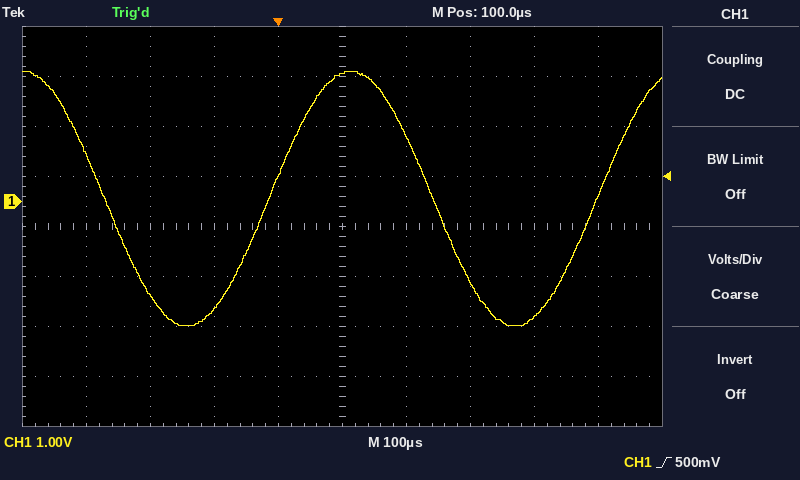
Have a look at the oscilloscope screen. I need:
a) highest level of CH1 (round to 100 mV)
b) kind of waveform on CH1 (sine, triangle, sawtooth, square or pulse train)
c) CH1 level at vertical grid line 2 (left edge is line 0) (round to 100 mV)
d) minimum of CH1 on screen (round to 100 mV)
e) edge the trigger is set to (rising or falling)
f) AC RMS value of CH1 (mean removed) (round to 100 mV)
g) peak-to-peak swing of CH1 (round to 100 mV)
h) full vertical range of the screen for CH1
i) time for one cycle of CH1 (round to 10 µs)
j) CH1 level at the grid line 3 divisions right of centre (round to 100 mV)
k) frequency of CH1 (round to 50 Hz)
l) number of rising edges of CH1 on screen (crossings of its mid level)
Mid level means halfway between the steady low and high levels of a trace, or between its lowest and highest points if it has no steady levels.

2.6 V
sine
-1.9 V
-2.5 V
rising
1.8 V
5.1 V
8 V
510 µs
-2.3 V
1.95 kHz
2
